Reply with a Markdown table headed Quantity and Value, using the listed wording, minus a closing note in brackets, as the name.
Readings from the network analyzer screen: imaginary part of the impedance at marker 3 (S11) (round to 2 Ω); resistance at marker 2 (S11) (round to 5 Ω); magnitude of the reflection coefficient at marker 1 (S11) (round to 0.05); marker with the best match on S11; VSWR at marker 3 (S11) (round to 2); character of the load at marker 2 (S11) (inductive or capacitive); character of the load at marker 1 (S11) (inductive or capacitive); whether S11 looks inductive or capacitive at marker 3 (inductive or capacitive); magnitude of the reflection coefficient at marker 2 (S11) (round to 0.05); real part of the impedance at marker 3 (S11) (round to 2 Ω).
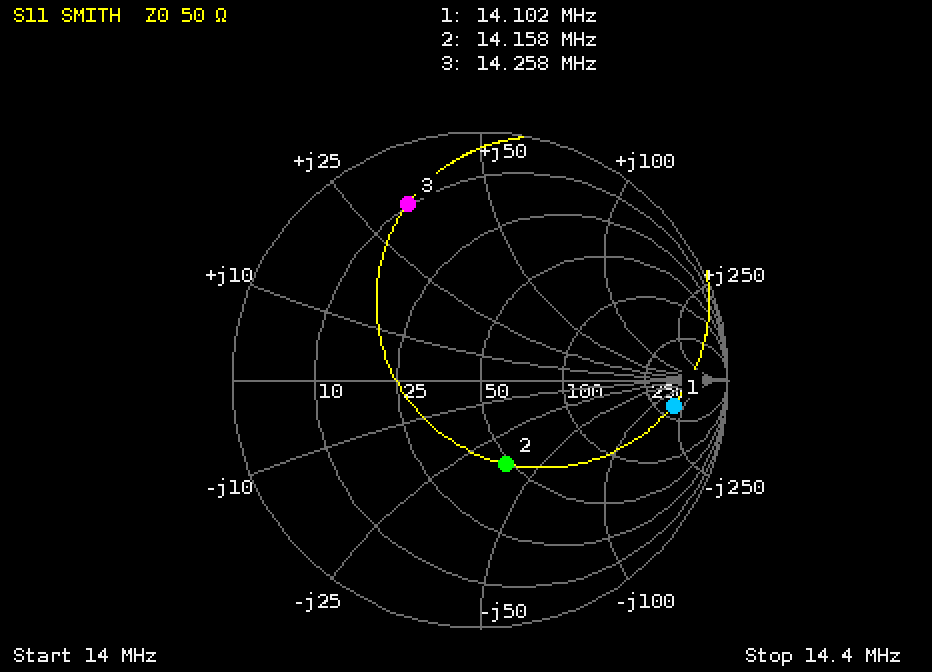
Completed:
| Quantity | Value |
|---|---|
| imaginary part of the impedance at marker 3 (S11) | +32 Ω |
| resistance at marker 2 (S11) | 50 Ω |
| magnitude of the reflection coefficient at marker 1 (S11) | 0.80 |
| marker with the best match on S11 | marker 2 |
| VSWR at marker 3 (S11) | 8 |
| character of the load at marker 2 (S11) | capacitive |
| character of the load at marker 1 (S11) | capacitive |
| whether S11 looks inductive or capacitive at marker 3 | inductive |
| magnitude of the reflection coefficient at marker 2 (S11) | 0.35 |
| real part of the impedance at marker 3 (S11) | 10 Ω |
